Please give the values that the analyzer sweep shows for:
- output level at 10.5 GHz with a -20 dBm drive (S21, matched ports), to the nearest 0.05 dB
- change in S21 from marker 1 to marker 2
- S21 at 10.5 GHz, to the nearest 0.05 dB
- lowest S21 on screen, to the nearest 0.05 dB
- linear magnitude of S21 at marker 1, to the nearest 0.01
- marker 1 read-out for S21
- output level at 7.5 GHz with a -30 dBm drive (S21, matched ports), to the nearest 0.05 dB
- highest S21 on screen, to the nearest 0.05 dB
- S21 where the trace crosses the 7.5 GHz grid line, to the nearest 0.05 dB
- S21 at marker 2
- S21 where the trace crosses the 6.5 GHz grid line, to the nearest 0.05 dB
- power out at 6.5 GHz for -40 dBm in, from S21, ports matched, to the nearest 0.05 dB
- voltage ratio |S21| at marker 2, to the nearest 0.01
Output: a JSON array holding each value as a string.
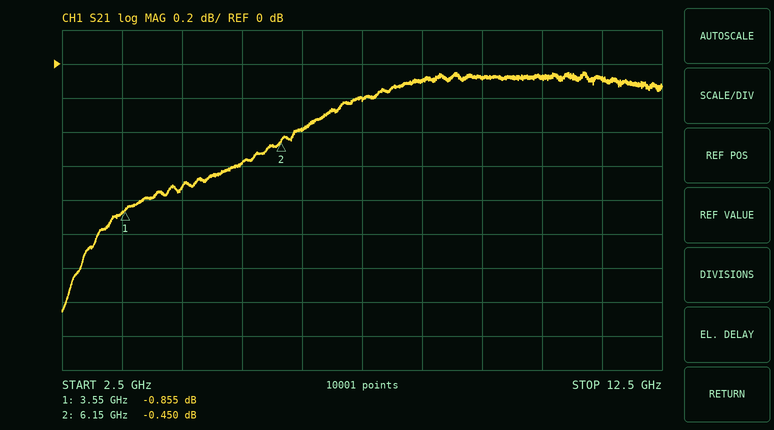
["-20.10 dBm", "0.405 dB", "-0.10 dB", "-1.45 dB", "0.91", "-0.855 dB", "-30.20 dBm", "-0.05 dB", "-0.20 dB", "-0.450 dB", "-0.40 dB", "-40.40 dBm", "0.95"]
